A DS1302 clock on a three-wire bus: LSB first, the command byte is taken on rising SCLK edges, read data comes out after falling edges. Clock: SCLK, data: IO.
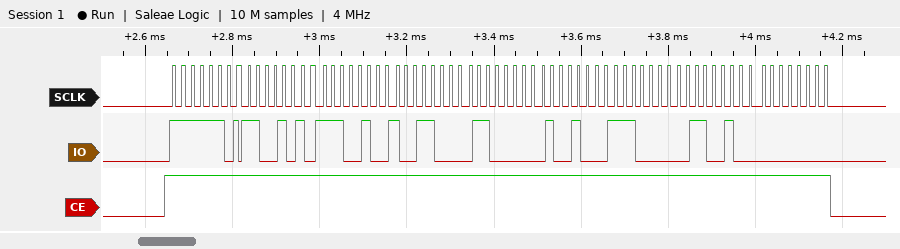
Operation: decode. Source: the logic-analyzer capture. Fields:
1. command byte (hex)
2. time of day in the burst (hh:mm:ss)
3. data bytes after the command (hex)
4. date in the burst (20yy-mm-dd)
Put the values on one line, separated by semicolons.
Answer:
0xBF; 19:27:53; 53 27 19 06 12 07 26 00; 2026-12-06
